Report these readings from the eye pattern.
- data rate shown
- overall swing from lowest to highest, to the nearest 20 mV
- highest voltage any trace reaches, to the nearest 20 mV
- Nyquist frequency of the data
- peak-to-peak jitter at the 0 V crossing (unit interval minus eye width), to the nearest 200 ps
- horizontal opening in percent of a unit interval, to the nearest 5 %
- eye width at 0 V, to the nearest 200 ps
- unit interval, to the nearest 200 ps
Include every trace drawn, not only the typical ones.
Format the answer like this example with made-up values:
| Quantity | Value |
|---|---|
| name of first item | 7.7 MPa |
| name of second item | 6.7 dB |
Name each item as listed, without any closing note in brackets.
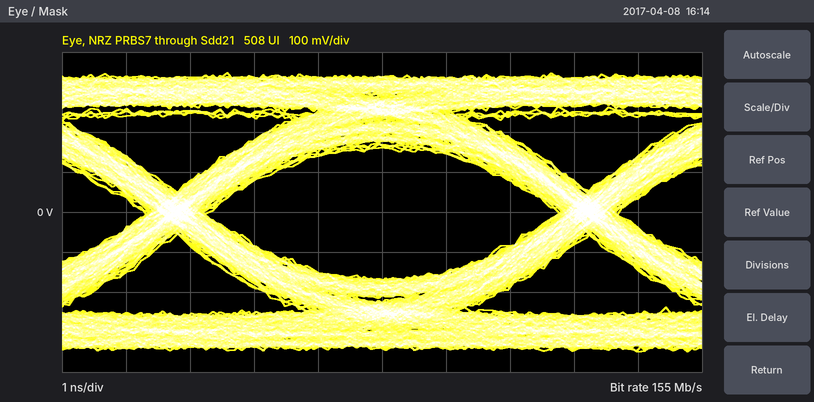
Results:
| Quantity | Value |
|---|---|
| data rate shown | 155 Mb/s |
| overall swing from lowest to highest, to the nearest 20 mV | 700 mV |
| highest voltage any trace reaches, to the nearest 20 mV | 340 mV |
| Nyquist frequency of the data | 77.5 MHz |
| peak-to-peak jitter at the 0 V crossing (unit interval minus eye width), to the nearest 200 ps | 1.0 ns |
| horizontal opening in percent of a unit interval, to the nearest 5 % | 85 % |
| eye width at 0 V, to the nearest 200 ps | 5.4 ns |
| unit interval, to the nearest 200 ps | 6.4 ns |
